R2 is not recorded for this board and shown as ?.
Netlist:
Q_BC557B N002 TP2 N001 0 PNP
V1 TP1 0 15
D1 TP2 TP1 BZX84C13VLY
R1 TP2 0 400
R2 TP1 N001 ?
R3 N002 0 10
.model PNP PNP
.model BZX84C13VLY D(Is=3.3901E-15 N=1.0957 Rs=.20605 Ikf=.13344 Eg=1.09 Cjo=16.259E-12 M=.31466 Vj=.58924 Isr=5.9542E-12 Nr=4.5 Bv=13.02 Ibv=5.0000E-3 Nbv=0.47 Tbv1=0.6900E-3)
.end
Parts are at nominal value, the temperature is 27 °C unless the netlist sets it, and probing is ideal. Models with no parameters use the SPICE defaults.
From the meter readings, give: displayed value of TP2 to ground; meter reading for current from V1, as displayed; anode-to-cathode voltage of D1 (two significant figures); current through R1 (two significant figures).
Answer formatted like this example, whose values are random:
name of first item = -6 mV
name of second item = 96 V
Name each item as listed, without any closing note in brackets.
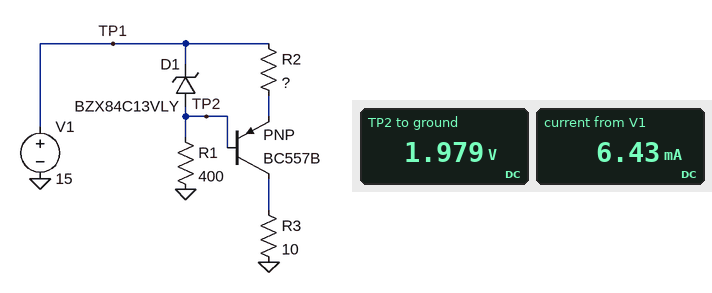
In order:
displayed value of TP2 to ground = 1.979 V
meter reading for current from V1, as displayed = 6.43 mA
anode-to-cathode voltage of D1 = -13 V
current through R1 = 4.9 mA
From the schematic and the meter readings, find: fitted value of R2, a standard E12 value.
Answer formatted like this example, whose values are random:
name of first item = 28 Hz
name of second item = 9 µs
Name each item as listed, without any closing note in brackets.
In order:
fitted value of R2, a standard E12 value = 8.2 kΩ
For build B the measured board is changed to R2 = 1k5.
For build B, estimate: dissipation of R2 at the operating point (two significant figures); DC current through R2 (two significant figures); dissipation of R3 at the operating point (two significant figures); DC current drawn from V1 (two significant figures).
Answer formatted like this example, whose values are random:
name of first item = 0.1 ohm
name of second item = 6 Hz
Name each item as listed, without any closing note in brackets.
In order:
dissipation of R2 at the operating point = 99 mW
DC current through R2 = 8.1 mA
dissipation of R3 at the operating point = 650 µW
DC current drawn from V1 = 13 mA
